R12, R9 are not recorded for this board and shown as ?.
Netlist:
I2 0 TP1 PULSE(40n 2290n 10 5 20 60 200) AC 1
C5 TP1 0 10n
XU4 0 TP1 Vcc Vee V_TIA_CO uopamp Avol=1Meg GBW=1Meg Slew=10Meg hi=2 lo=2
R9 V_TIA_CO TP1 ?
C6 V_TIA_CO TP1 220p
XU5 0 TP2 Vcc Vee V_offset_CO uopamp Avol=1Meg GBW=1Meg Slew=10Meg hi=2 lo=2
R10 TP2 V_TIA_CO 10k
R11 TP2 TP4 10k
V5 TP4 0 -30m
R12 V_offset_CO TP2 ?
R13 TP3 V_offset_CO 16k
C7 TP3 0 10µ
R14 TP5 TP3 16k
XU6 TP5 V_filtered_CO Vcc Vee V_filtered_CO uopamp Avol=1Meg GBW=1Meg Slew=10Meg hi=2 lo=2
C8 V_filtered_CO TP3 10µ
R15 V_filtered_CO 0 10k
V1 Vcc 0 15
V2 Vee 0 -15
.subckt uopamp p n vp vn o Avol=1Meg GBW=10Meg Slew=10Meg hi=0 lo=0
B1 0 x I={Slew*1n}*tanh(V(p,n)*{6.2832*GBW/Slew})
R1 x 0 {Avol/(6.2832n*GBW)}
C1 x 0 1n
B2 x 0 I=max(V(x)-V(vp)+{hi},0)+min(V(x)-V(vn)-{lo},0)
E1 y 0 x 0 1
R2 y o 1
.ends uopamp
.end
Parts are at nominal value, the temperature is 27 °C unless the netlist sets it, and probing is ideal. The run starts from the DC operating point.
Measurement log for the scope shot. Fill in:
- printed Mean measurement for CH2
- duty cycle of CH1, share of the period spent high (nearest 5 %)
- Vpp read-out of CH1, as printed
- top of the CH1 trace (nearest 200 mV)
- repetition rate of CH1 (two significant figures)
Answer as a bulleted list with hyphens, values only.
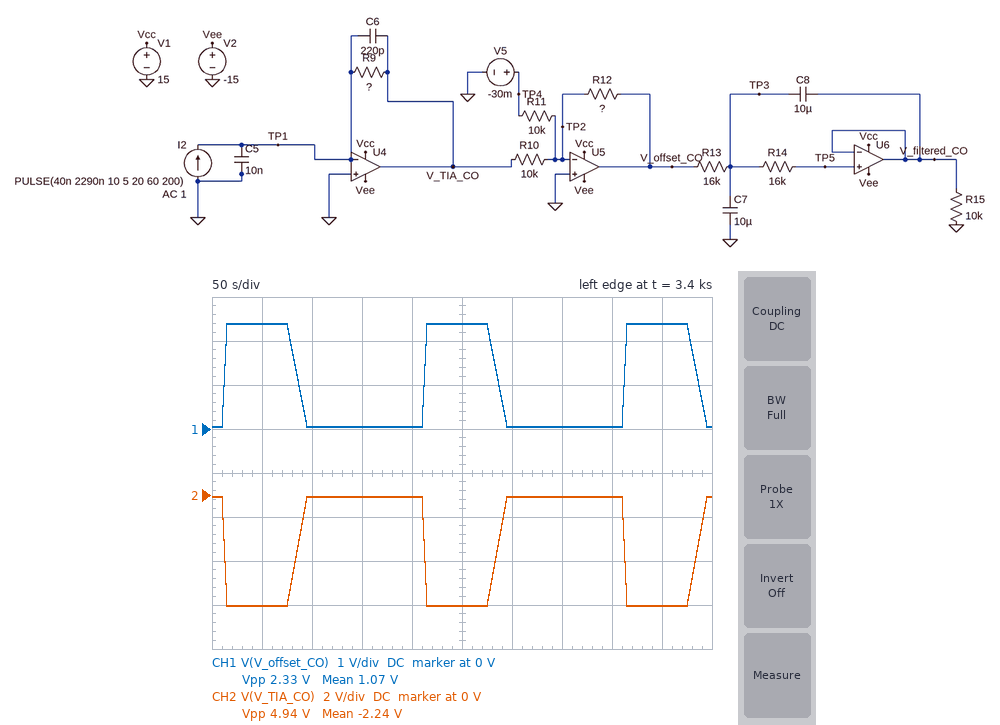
- -2.24 V
- 35 %
- 2.33 V
- 2.4 V
- 5.0 mHz
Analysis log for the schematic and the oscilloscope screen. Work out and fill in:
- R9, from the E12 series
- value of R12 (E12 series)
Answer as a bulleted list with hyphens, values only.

- 2.2 MΩ
- 4.7 kΩ
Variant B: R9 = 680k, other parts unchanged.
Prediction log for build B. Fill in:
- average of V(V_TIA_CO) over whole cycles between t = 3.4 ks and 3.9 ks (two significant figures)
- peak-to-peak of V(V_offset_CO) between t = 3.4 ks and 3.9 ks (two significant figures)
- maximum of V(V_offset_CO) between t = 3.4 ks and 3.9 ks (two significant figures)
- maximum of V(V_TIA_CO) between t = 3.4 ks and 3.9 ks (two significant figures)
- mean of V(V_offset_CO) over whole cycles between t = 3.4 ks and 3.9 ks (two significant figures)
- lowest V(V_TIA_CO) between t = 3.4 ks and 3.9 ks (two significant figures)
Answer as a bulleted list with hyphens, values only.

- -580 mV
- 720 mV
- 750 mV
- -27 mV
- 290 mV
- -1.6 V
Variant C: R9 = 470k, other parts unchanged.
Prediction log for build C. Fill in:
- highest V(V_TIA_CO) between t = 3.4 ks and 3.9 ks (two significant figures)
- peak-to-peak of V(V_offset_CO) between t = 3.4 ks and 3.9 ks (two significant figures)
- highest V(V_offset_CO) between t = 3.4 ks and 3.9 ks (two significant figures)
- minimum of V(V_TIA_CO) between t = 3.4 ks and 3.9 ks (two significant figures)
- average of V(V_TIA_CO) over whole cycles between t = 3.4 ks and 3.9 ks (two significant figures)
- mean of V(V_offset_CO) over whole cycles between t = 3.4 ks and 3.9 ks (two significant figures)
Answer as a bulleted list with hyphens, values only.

- -19 mV
- 500 mV
- 520 mV
- -1.1 V
- -400 mV
- 200 mV
